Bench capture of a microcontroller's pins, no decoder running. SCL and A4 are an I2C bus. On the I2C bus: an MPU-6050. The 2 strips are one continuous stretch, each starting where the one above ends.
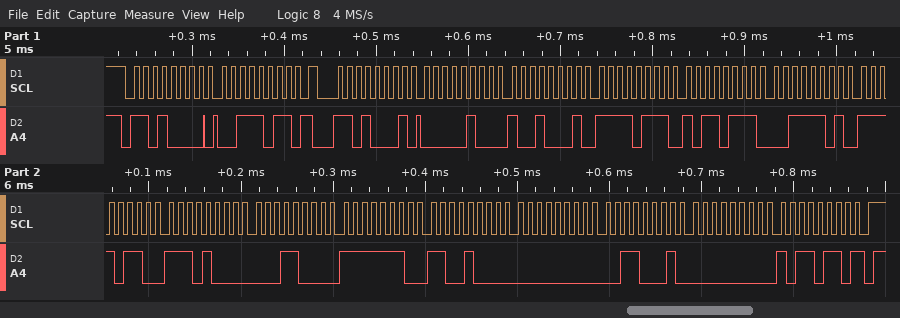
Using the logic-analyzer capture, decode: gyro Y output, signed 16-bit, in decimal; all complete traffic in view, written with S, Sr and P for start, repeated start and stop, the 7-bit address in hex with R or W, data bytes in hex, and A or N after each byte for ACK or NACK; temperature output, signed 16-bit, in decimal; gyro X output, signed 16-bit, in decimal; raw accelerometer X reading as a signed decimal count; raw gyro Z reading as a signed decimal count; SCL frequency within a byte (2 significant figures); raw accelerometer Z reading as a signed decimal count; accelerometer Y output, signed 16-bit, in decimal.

49
S 68W A 3B A Sr 68R A 04 A 91 A F7 A B7 A 3D A F6 A E8 A 18 A FE A C8 A 00 A 31 A 00 A B6 N P
-6120
-312
1169
182
100 kHz
15862
-2121
